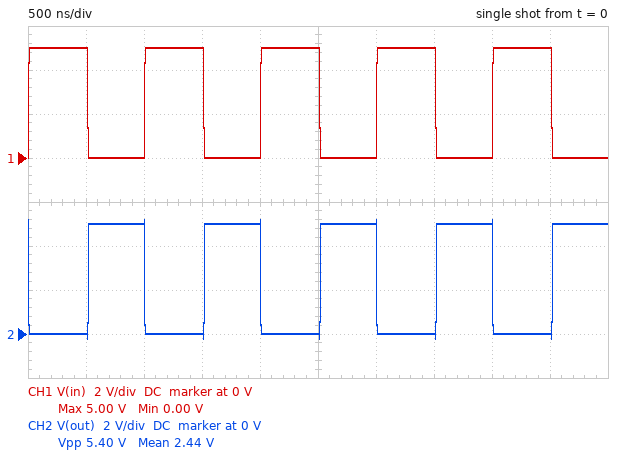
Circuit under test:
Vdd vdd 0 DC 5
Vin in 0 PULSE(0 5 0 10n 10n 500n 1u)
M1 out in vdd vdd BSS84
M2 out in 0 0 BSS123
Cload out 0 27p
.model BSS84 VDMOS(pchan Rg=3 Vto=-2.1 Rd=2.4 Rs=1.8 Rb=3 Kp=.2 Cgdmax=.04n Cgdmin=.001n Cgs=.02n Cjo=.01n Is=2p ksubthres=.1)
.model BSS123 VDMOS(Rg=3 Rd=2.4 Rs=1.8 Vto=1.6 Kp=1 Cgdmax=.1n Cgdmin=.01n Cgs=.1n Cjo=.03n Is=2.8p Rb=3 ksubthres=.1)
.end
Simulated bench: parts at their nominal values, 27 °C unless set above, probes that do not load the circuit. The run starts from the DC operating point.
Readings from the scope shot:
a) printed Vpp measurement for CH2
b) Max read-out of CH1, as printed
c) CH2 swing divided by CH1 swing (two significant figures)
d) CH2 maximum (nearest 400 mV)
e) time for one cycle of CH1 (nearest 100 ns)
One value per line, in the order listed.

5.40 V
5.00 V
1.1
5.2 V
1.0 µs
